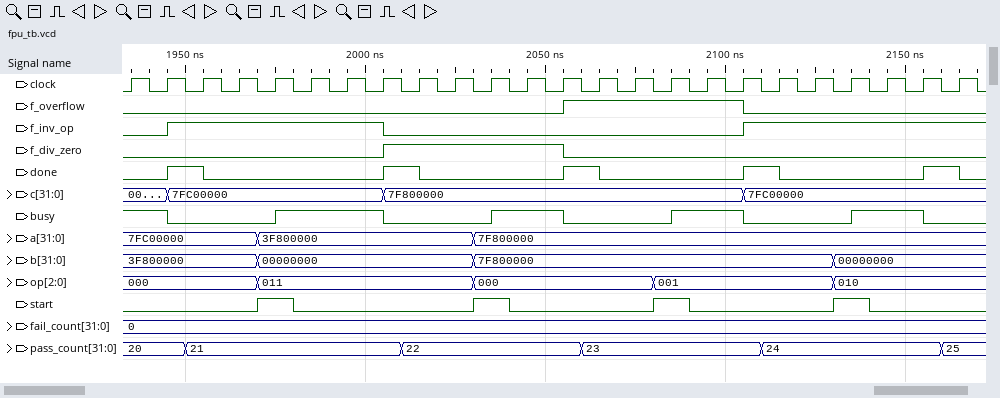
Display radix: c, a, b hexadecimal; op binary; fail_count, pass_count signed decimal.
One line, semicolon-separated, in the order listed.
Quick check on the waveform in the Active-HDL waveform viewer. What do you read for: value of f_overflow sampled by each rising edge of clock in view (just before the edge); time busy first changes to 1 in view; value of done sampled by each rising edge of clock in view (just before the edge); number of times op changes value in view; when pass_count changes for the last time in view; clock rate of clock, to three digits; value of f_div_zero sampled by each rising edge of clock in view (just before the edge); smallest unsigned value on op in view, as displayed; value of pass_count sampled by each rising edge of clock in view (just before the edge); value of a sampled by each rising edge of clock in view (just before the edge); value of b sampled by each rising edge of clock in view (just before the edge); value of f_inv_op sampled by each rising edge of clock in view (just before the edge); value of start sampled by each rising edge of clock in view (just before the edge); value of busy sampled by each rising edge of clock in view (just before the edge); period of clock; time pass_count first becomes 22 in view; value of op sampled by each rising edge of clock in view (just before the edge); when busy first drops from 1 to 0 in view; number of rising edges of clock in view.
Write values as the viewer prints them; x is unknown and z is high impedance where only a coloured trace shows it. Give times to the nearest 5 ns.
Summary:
0 0 0 0 0 0 0 0 0 0 0 0 0 1 1 1 1 1 0 0 0 0 0 0; 1975 ns; 0 0 1 0 0 0 0 0 1 0 0 0 0 1 0 0 0 0 1 0 0 0 0 1; 4; 2160 ns; 100 MHz; 0 0 0 0 0 0 0 0 1 1 1 1 1 0 0 0 0 0 0 0 0 0 0 0; 000; 20, 20, 21, 21, 21, 21, 21, 21, 22, 22, 22, 22, 22, 23, 23, 23, 23, 23, 24, 24, 24, 24, 24, 25; 7FC00000, 7FC00000, 7FC00000, 7FC00000, 3F800000, 3F800000, 3F800000, 3F800000, 3F800000, 3F800000, 7F800000, 7F800000, 7F800000, 7F800000, 7F800000, 7F800000, 7F800000, 7F800000, 7F800000, 7F800000, 7F800000, 7F800000, 7F800000, 7F800000; 3F800000, 3F800000, 3F800000, 3F800000, 00000000, 00000000, 00000000, 00000000, 00000000, 00000000, 7F800000, 7F800000, 7F800000, 7F800000, 7F800000, 7F800000, 7F800000, 7F800000, 7F800000, 7F800000, 00000000, 00000000, 00000000, 00000000; 0 0 1 1 1 1 1 1 0 0 0 0 0 0 0 0 0 0 1 1 1 1 1 1; 0 0 0 0 1 0 0 0 0 0 1 0 0 0 0 1 0 0 0 0 1 0 0 0; 1 1 0 0 0 1 1 1 0 0 0 1 1 0 0 0 1 1 0 0 0 1 1 0; 10 ns; 2010 ns; 000, 000, 000, 000, 011, 011, 011, 011, 011, 011, 000, 000, 000, 000, 000, 001, 001, 001, 001, 001, 010, 010, 010, 010; 1945 ns; 24
